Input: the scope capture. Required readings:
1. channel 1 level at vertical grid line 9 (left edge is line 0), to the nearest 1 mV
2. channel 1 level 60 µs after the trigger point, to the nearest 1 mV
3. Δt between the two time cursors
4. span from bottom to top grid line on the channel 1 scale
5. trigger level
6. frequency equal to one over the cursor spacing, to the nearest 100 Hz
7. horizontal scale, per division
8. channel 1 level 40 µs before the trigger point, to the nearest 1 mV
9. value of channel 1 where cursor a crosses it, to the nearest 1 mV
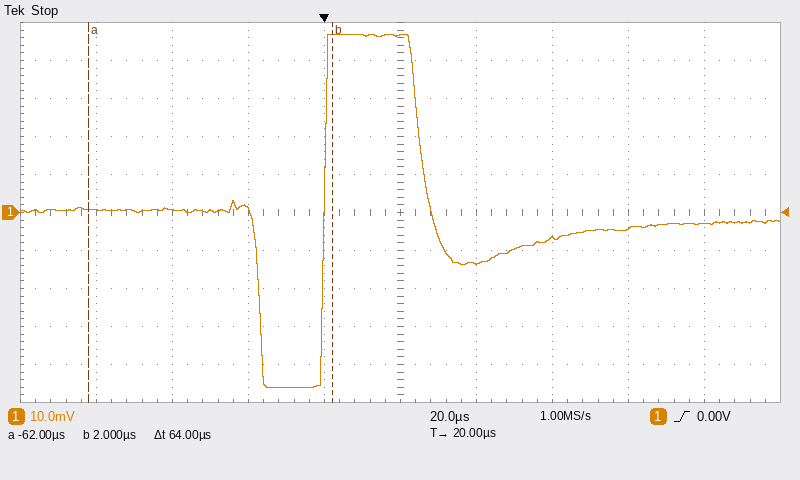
-3 mV
-7 mV
64 µs
100 mV
0.00 V
15.6 kHz
20 µs
1 mV
1 mV
